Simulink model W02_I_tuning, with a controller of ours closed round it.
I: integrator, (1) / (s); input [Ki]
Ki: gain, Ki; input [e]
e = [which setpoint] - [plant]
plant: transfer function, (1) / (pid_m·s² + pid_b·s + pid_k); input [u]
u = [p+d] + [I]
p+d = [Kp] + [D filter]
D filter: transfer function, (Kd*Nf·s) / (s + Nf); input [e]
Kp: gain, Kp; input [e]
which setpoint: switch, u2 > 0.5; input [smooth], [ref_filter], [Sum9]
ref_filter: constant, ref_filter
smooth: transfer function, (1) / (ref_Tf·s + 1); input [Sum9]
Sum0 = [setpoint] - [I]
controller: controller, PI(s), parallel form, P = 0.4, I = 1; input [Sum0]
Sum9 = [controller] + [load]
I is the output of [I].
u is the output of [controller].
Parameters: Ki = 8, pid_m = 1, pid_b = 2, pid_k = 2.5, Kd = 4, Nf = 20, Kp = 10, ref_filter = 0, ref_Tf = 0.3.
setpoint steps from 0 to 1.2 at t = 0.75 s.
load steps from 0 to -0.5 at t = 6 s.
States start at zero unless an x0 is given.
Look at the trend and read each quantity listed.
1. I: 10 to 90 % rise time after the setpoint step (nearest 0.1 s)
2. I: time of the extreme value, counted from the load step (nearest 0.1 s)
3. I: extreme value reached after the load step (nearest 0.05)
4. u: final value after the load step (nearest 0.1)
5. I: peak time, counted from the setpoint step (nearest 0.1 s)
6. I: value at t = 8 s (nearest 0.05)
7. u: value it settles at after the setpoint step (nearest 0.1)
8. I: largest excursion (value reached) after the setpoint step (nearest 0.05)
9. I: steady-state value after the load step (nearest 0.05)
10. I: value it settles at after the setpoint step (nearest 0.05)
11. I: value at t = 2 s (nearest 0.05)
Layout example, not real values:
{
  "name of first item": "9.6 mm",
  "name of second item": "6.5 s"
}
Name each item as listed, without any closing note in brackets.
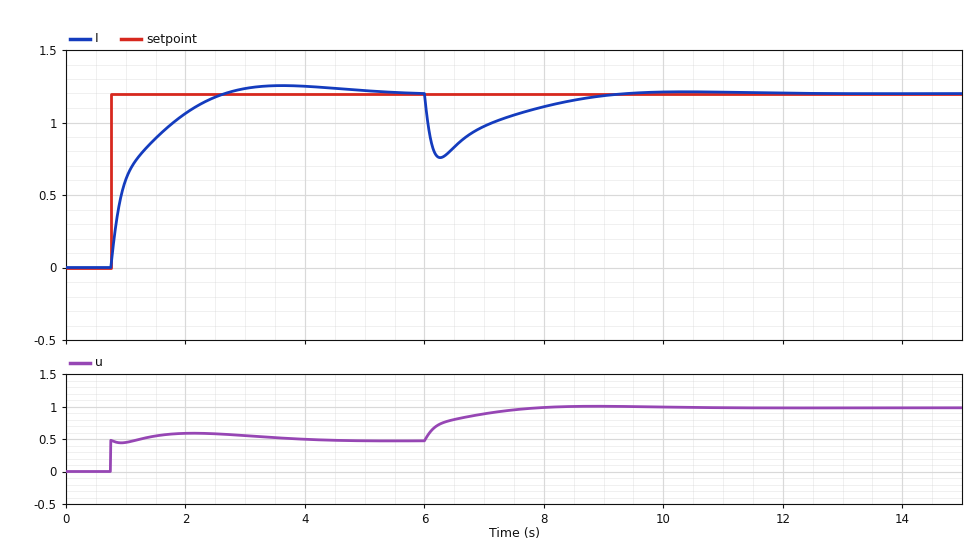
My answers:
{
  "I: 10 to 90 % rise time after the setpoint step": "1.3 s",
  "I: time of the extreme value, counted from the load step": "0.3 s",
  "I: extreme value reached after the load step": "0.75",
  "u: final value after the load step": "1.0",
  "I: peak time, counted from the setpoint step": "2.9 s",
  "I: value at t = 8 s": "1.10",
  "u: value it settles at after the setpoint step": "0.5",
  "I: largest excursion (value reached) after the setpoint step": "1.25",
  "I: steady-state value after the load step": "1.20",
  "I: value it settles at after the setpoint step": "1.20",
  "I: value at t = 2 s": "1.05"
}
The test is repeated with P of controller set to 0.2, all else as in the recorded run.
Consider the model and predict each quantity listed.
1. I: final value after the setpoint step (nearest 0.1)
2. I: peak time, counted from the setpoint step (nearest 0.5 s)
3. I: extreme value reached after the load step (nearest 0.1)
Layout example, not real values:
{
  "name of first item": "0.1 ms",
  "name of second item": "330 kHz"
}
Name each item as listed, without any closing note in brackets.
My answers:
{
  "I: final value after the setpoint step": "1.2",
  "I: peak time, counted from the setpoint step": "2.5 s",
  "I: extreme value reached after the load step": "0.7"
}
